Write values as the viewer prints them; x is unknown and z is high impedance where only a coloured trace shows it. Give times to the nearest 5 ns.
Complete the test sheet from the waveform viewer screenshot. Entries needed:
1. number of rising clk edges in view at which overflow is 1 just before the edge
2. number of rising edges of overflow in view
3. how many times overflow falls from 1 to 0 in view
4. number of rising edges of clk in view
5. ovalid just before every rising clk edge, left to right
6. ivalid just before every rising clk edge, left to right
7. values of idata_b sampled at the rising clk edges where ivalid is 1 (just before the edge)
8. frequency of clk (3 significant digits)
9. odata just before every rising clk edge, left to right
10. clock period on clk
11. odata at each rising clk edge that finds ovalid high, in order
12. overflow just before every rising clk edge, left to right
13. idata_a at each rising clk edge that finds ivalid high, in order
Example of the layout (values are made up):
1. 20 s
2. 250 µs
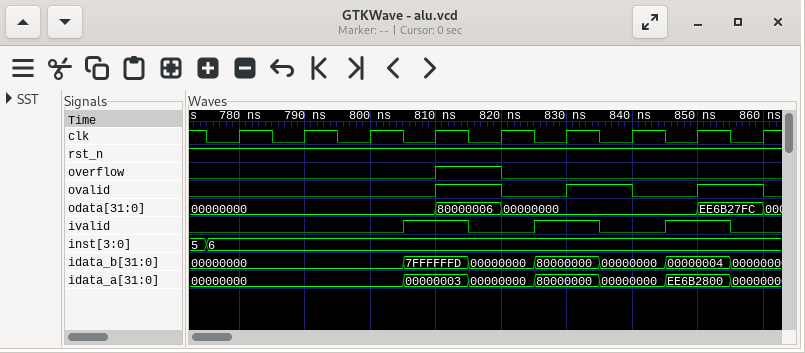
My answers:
1. 1
2. 1
3. 1
4. 9
5. 0 0 0 0 1 0 1 0 1
6. 0 0 0 1 0 1 0 1 0
7. 7FFFFFFD, 80000000, 00000004
8. 100 MHz
9. 00000000, 00000000, 00000000, 00000000, 80000006, 00000000, 00000000, 00000000, EE6B27FC
10. 10 ns
11. 80000006, 00000000, EE6B27FC
12. 0 0 0 0 1 0 0 0 0
13. 00000003, 80000000, EE6B2800
